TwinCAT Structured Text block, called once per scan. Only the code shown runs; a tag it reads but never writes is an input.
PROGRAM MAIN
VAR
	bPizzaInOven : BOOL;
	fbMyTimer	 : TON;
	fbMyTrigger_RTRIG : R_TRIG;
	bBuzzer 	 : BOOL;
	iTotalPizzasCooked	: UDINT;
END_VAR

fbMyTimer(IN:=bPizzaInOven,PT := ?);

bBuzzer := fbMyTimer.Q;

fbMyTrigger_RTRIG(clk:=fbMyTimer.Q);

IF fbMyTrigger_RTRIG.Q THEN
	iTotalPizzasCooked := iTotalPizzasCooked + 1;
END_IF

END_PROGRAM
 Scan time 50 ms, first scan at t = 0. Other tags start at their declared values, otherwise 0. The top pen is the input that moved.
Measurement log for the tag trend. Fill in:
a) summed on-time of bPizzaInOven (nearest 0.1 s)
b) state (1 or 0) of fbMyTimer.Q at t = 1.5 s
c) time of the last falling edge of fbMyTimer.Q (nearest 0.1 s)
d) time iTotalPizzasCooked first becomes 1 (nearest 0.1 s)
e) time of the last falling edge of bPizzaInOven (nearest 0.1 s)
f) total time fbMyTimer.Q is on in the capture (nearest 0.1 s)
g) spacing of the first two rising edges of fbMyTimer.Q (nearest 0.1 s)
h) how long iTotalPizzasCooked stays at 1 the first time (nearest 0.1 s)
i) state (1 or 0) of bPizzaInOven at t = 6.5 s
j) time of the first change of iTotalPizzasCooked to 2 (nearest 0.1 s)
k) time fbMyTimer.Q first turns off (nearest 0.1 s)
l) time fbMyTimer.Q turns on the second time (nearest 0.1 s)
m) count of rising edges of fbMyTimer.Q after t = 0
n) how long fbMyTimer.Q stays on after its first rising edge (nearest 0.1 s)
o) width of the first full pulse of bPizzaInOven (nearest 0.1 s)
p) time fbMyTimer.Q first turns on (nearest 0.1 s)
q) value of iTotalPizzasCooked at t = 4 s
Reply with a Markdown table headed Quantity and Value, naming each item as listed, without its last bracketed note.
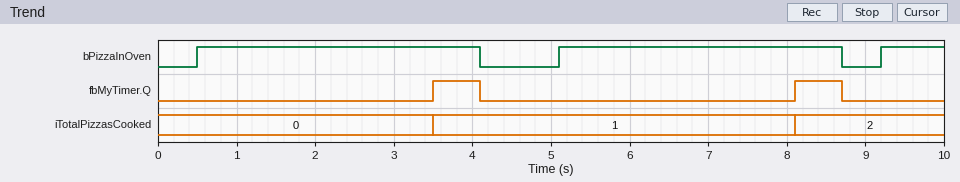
| Quantity | Value |
|---|---|
| summed on-time of bPizzaInOven | 8.0 s |
| state (1 or 0) of fbMyTimer.Q at t = 1.5 s | 0 |
| time of the last falling edge of fbMyTimer.Q | 8.7 s |
| time iTotalPizzasCooked first becomes 1 | 3.5 s |
| time of the last falling edge of bPizzaInOven | 8.7 s |
| total time fbMyTimer.Q is on in the capture | 1.2 s |
| spacing of the first two rising edges of fbMyTimer.Q | 4.6 s |
| how long iTotalPizzasCooked stays at 1 the first time | 4.6 s |
| state (1 or 0) of bPizzaInOven at t = 6.5 s | 1 |
| time of the first change of iTotalPizzasCooked to 2 | 8.1 s |
| time fbMyTimer.Q first turns off | 4.1 s |
| time fbMyTimer.Q turns on the second time | 8.1 s |
| count of rising edges of fbMyTimer.Q after t = 0 | 2 |
| how long fbMyTimer.Q stays on after its first rising edge | 0.6 s |
| width of the first full pulse of bPizzaInOven | 3.6 s |
| time fbMyTimer.Q first turns on | 3.5 s |
| value of iTotalPizzasCooked at t = 4 s | 1 |
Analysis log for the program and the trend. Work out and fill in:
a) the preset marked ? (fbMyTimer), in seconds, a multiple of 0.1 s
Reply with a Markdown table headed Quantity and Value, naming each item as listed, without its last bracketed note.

| Quantity | Value |
|---|---|
| the preset marked ? (fbMyTimer), in seconds, a multiple of 0.1 s | 3.0 s |
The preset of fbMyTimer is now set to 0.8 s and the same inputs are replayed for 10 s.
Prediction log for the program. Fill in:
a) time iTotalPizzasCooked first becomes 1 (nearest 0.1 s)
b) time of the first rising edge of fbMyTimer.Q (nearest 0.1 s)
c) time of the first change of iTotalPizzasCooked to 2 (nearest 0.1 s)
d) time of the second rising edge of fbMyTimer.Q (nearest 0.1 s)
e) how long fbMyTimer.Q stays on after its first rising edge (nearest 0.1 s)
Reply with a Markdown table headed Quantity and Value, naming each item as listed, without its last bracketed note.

| Quantity | Value |
|---|---|
| time iTotalPizzasCooked first becomes 1 | 1.3 s |
| time of the first rising edge of fbMyTimer.Q | 1.3 s |
| time of the first change of iTotalPizzasCooked to 2 | 5.9 s |
| time of the second rising edge of fbMyTimer.Q | 5.9 s |
| how long fbMyTimer.Q stays on after its first rising edge | 2.8 s |
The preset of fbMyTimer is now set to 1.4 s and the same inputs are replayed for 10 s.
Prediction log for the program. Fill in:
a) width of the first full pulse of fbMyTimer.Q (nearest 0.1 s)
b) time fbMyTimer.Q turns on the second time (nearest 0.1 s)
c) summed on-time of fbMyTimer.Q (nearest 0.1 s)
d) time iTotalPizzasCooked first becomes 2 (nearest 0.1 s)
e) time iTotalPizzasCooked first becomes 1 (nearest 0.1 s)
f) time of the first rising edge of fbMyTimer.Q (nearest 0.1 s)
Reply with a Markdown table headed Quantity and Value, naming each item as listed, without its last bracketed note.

| Quantity | Value |
|---|---|
| width of the first full pulse of fbMyTimer.Q | 2.2 s |
| time fbMyTimer.Q turns on the second time | 6.5 s |
| summed on-time of fbMyTimer.Q | 4.4 s |
| time iTotalPizzasCooked first becomes 2 | 6.5 s |
| time iTotalPizzasCooked first becomes 1 | 1.9 s |
| time of the first rising edge of fbMyTimer.Q | 1.9 s |
